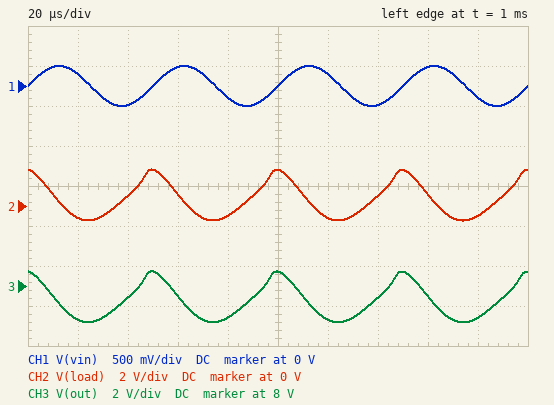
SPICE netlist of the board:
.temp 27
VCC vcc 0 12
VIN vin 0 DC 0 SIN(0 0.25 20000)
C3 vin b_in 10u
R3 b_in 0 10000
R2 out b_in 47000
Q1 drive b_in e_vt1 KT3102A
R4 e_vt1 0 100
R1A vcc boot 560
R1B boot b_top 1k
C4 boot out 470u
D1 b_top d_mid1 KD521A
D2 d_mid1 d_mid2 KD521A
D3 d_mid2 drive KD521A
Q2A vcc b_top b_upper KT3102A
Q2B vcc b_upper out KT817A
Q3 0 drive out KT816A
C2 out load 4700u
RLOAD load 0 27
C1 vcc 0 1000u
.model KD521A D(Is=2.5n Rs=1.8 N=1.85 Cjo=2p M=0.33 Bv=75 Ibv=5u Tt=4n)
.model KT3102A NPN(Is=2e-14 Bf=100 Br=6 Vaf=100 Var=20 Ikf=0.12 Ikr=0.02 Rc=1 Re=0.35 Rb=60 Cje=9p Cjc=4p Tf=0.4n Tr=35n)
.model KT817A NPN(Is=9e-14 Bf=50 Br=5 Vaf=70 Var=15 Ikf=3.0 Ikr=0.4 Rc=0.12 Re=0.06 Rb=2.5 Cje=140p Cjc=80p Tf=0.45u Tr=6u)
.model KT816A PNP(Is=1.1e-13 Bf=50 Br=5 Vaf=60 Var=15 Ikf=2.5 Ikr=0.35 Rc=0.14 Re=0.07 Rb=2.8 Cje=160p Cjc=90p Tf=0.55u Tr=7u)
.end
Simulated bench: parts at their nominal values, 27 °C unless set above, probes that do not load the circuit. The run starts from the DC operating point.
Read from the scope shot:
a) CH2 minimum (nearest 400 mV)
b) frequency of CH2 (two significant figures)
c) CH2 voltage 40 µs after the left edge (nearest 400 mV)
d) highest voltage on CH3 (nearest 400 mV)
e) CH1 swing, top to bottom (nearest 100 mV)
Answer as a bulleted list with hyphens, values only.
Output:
- -800 mV
- 20 kHz
- 400 mV
- 8.8 V
- 500 mV
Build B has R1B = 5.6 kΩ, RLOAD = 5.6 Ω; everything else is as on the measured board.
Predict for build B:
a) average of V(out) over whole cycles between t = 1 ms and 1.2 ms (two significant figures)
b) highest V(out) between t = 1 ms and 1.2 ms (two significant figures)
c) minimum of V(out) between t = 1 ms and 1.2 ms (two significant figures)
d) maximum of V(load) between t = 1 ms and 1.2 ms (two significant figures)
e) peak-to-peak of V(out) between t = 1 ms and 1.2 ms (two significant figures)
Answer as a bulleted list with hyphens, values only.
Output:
- 5.6 V
- 6.8 V
- 5.1 V
- 2.0 V
- 1.7 V
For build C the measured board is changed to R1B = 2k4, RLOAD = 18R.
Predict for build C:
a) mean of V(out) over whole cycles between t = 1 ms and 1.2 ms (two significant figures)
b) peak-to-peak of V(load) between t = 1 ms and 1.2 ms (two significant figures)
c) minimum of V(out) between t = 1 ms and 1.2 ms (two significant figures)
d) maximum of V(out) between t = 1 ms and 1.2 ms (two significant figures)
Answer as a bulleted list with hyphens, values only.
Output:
- 7.8 V
- 4.8 V
- 6.3 V
- 11 V
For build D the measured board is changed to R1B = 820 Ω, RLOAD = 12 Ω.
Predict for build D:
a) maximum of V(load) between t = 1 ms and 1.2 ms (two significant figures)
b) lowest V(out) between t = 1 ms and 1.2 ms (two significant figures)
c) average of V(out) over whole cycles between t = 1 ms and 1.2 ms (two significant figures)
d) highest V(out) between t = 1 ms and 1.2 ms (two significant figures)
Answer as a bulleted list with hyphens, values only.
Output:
- 670 mV
- 6.8 V
- 7.2 V
- 7.8 V
